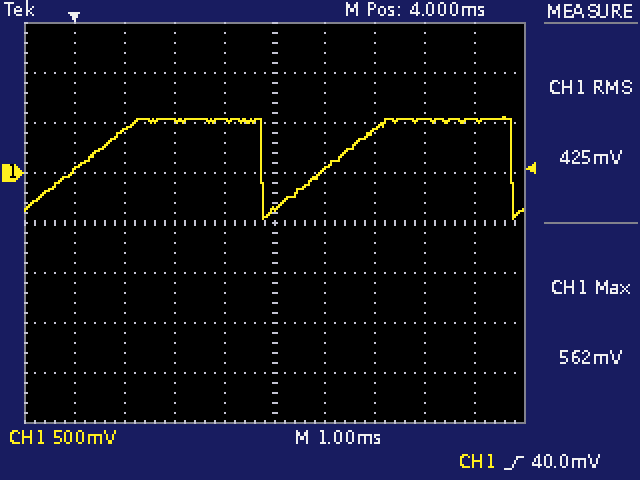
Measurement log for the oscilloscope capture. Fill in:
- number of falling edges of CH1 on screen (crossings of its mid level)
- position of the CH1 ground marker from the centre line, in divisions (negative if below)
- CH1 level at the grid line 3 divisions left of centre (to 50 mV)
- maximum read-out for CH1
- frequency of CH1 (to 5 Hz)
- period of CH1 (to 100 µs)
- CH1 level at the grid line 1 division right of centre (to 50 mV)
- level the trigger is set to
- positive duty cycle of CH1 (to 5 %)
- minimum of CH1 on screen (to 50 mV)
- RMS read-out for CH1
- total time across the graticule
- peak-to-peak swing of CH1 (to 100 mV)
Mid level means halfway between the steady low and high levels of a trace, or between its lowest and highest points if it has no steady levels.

2
+1.0 div
450 mV
562 mV
200 Hz
5.0 ms
50 mV
40.0 mV
75 %
-450 mV
425 mV
10 ms
1.00 V
